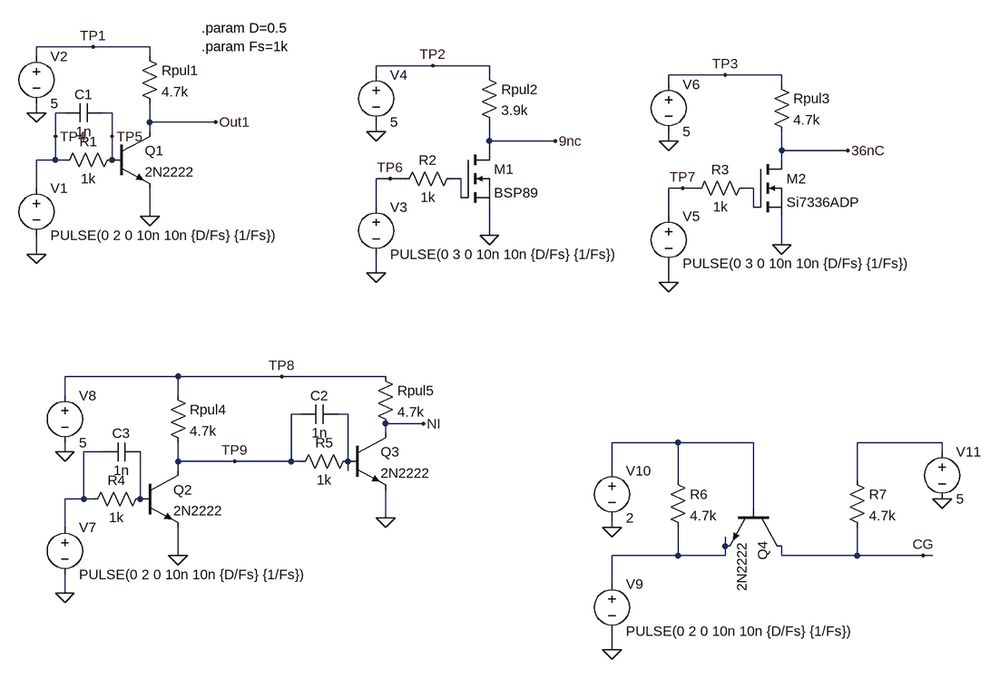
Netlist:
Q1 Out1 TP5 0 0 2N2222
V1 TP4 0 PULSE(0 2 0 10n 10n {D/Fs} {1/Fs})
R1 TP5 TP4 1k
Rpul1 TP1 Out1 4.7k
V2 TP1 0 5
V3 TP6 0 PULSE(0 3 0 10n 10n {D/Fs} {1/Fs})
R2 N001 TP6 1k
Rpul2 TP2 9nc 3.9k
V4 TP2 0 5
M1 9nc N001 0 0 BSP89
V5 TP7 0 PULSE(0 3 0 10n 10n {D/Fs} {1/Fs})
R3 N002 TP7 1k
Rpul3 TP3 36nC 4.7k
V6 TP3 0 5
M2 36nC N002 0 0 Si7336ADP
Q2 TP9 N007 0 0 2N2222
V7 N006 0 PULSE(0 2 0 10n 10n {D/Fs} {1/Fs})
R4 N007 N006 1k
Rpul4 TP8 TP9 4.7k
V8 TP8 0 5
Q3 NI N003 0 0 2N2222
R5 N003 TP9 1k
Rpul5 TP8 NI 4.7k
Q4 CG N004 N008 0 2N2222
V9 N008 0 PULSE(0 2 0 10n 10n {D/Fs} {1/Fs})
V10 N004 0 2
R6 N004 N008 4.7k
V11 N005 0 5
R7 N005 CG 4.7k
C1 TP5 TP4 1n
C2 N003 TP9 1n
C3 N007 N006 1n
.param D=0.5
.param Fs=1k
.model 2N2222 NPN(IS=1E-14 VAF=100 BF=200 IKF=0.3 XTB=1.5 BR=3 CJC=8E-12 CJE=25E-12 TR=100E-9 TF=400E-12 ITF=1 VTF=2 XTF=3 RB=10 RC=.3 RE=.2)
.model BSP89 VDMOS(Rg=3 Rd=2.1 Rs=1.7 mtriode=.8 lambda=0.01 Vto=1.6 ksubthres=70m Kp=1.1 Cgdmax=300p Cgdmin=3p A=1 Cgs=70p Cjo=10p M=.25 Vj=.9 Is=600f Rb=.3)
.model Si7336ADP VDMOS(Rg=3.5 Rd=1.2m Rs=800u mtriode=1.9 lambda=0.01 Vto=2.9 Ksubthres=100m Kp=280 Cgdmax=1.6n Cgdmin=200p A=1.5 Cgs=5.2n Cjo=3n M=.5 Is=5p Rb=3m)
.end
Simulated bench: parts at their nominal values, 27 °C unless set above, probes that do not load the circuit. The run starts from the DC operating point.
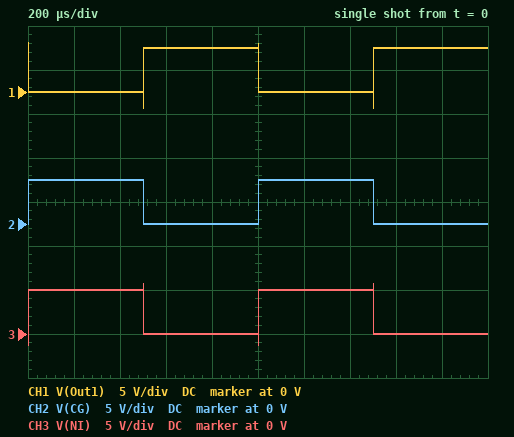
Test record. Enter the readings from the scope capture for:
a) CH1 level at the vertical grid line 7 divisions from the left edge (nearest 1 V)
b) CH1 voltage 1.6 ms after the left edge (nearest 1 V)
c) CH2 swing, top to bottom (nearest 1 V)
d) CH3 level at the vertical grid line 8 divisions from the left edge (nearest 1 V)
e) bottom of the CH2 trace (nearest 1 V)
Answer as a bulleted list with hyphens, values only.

- 0 V
- 5 V
- 5 V
- 0 V
- 0 V
